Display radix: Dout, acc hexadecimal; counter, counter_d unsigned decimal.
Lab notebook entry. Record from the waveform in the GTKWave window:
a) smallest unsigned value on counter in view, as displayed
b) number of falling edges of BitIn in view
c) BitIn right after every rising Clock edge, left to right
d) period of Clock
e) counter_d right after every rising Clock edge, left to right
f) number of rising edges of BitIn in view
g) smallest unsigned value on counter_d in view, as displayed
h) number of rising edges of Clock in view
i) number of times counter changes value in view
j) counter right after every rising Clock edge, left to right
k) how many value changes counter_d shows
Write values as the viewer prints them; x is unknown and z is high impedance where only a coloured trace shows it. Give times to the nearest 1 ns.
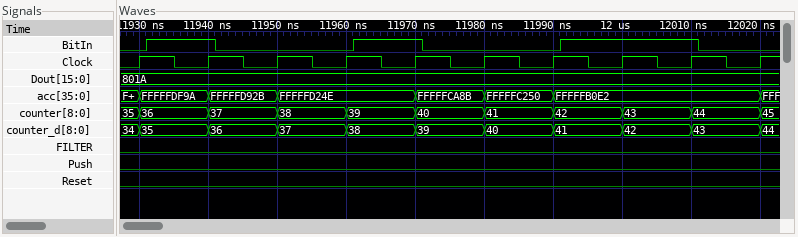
35
3
0 1 0 0 1 0 0 1 1 0
10 ns
35, 36, 37, 38, 39, 40, 41, 42, 43, 44
3
34
10
10
36, 37, 38, 39, 40, 41, 42, 43, 44, 45
10
